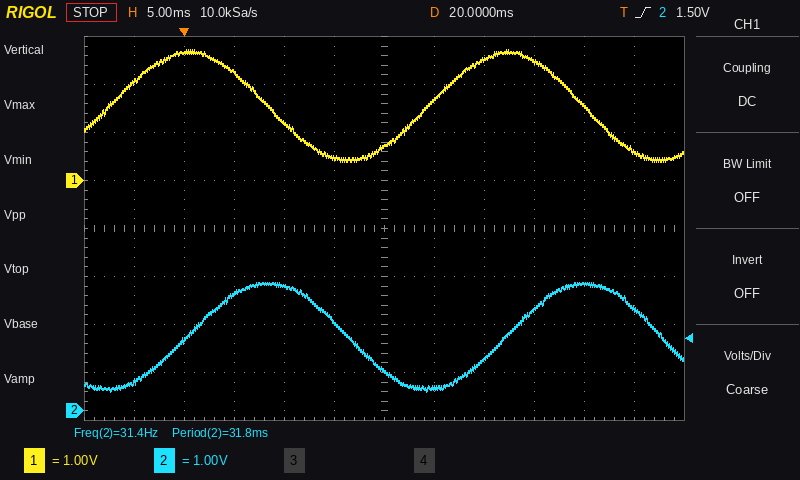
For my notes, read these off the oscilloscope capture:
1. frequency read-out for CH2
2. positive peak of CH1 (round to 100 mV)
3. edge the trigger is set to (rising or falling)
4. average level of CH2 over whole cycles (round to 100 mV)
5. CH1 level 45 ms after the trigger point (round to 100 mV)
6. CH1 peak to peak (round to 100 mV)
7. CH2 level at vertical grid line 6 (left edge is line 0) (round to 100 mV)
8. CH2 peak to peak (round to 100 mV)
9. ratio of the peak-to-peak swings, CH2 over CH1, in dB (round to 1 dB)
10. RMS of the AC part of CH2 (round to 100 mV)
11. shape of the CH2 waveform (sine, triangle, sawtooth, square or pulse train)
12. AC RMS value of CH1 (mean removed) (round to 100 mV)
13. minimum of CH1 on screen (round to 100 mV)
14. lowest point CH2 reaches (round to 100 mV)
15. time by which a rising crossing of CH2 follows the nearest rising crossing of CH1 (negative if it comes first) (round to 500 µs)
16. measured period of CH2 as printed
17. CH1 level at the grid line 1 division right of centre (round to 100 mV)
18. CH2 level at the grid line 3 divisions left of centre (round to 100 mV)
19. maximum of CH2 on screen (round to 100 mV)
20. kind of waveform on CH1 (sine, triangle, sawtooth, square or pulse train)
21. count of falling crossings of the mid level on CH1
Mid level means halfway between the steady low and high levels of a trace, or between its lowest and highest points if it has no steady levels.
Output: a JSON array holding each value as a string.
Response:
["31.4 Hz", "2.7 V", "rising", "1.6 V", "600 mV", "2.3 V", "800 mV", "2.3 V", "0 dB", "800 mV", "sine", "800 mV", "400 mV", "400 mV", "+7.5 ms", "31.8 ms", "1.7 V", "2.4 V", "2.7 V", "sine", "2"]
